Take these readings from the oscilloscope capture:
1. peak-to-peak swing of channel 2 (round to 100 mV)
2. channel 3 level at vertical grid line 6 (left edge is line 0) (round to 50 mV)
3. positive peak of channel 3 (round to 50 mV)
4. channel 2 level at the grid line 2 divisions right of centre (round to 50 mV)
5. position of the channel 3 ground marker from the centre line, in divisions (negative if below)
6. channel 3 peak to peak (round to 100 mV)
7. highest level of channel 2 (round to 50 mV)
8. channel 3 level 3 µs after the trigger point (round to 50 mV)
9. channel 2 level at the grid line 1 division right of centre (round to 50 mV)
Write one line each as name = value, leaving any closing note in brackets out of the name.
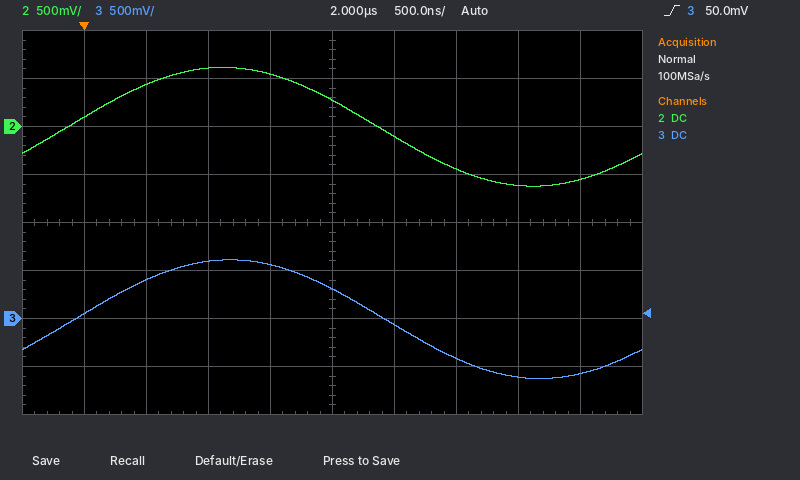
peak-to-peak swing of channel 2 = 1.20 V
channel 3 level at vertical grid line 6 (left edge is line 0) = -50 mV
positive peak of channel 3 = 600 mV
channel 2 level at the grid line 2 divisions right of centre = -450 mV
position of the channel 3 ground marker from the centre line, in divisions = -2.0 div
channel 3 peak to peak = 1.20 V
highest level of channel 2 = 600 mV
channel 3 level 3 µs after the trigger point = -400 mV
channel 2 level at the grid line 1 division right of centre = -100 mV
